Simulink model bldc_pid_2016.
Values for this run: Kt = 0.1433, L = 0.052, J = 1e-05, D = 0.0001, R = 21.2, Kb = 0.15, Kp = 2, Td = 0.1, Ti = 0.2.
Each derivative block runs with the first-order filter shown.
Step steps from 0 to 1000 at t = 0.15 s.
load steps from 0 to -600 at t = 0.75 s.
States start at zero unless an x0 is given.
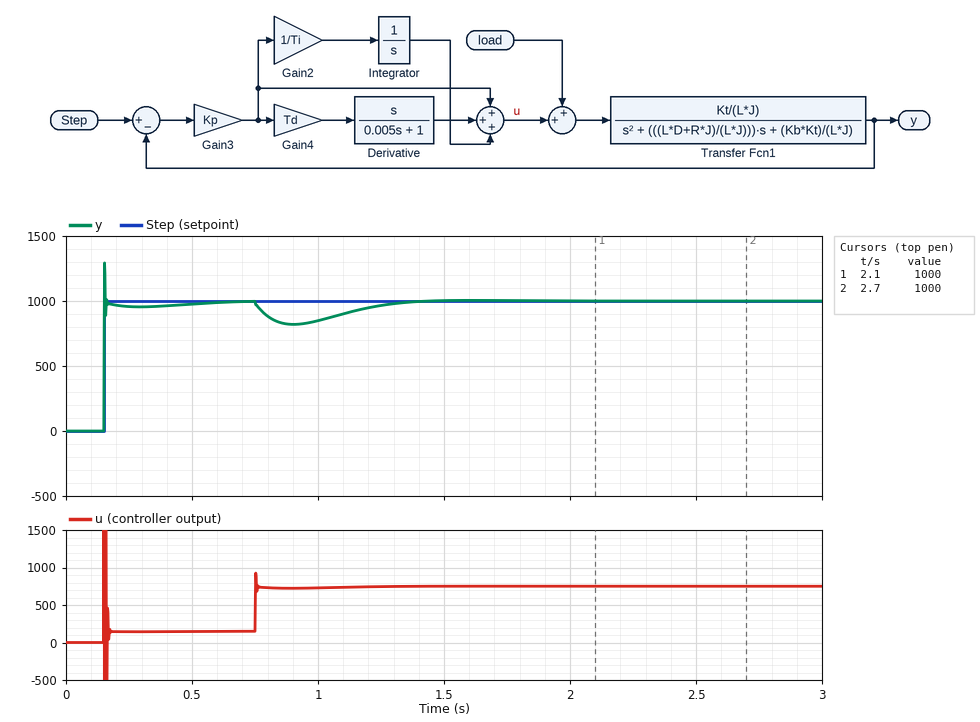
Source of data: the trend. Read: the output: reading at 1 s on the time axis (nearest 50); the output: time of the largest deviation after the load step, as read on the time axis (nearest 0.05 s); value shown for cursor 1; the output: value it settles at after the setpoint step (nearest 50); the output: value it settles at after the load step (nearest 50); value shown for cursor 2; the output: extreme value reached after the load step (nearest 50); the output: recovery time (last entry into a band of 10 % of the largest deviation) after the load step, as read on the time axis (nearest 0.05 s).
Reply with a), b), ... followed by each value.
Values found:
a) 850
b) 0.90 s
c) 1000
d) 1000
e) 1000
f) 1000
g) 800
h) 1.30 s
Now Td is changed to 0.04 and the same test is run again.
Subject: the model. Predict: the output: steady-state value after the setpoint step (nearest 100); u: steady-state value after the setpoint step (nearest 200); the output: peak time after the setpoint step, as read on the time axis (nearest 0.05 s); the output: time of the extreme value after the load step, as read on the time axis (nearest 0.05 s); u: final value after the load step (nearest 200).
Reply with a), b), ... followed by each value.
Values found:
a) 1000
b) 200
c) 0.15 s
d) 0.85 s
e) 800
